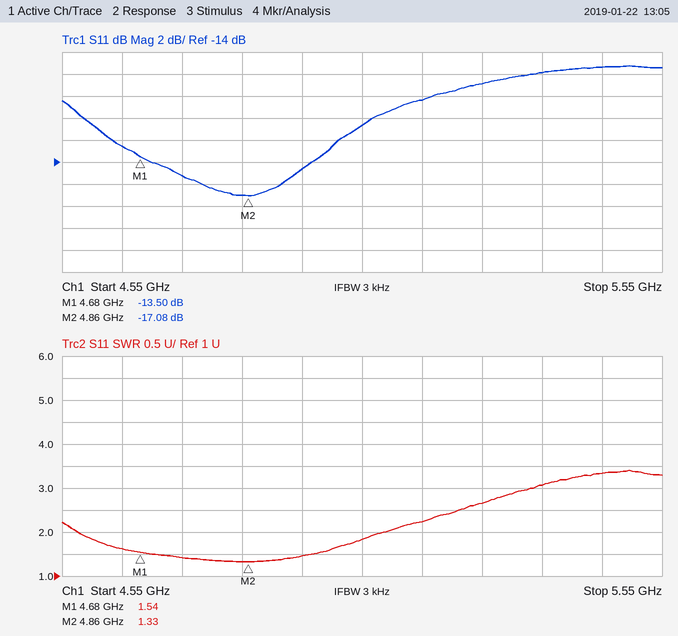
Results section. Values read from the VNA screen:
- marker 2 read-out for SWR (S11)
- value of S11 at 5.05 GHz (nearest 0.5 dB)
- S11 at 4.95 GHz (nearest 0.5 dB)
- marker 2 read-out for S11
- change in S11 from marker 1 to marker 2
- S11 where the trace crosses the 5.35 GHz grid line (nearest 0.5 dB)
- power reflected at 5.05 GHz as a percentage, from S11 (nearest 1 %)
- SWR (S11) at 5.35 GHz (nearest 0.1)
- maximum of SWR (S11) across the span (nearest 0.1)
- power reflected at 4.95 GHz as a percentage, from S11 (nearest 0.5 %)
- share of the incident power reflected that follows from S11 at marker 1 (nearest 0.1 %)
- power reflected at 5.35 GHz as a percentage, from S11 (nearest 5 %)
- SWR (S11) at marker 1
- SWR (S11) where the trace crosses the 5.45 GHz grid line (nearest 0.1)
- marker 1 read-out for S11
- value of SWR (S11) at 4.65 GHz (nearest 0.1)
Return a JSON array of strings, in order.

["1.33", "-10.5 dB", "-14.5 dB", "-17.08 dB", "-3.58 dB", "-6.0 dB", "9 %", "3.1", "3.4", "3.5 %", "4.5 %", "25 %", "1.54", "3.3", "-13.50 dB", "1.6"]
